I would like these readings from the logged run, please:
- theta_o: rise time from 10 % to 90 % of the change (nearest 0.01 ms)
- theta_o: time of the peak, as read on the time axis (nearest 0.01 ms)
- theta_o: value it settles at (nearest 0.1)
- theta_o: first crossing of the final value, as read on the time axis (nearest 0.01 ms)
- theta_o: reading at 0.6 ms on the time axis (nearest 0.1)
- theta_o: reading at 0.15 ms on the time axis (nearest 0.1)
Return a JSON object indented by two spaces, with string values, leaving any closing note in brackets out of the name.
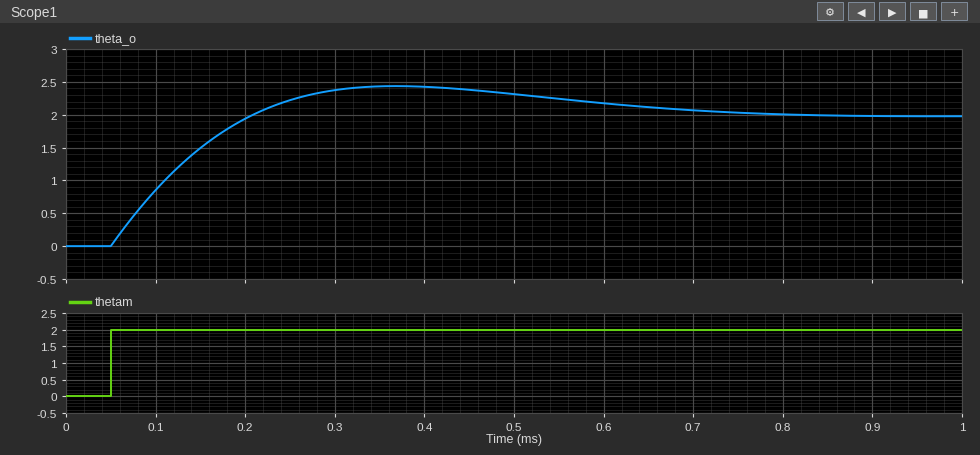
{
  "theta_o: rise time from 10 % to 90 % of the change": "0.12 ms",
  "theta_o: time of the peak, as read on the time axis": "0.37 ms",
  "theta_o: value it settles at": "2.0",
  "theta_o: first crossing of the final value, as read on the time axis": "0.21 ms",
  "theta_o: reading at 0.6 ms on the time axis": "2.2",
  "theta_o: reading at 0.15 ms on the time axis": "1.5"
}
